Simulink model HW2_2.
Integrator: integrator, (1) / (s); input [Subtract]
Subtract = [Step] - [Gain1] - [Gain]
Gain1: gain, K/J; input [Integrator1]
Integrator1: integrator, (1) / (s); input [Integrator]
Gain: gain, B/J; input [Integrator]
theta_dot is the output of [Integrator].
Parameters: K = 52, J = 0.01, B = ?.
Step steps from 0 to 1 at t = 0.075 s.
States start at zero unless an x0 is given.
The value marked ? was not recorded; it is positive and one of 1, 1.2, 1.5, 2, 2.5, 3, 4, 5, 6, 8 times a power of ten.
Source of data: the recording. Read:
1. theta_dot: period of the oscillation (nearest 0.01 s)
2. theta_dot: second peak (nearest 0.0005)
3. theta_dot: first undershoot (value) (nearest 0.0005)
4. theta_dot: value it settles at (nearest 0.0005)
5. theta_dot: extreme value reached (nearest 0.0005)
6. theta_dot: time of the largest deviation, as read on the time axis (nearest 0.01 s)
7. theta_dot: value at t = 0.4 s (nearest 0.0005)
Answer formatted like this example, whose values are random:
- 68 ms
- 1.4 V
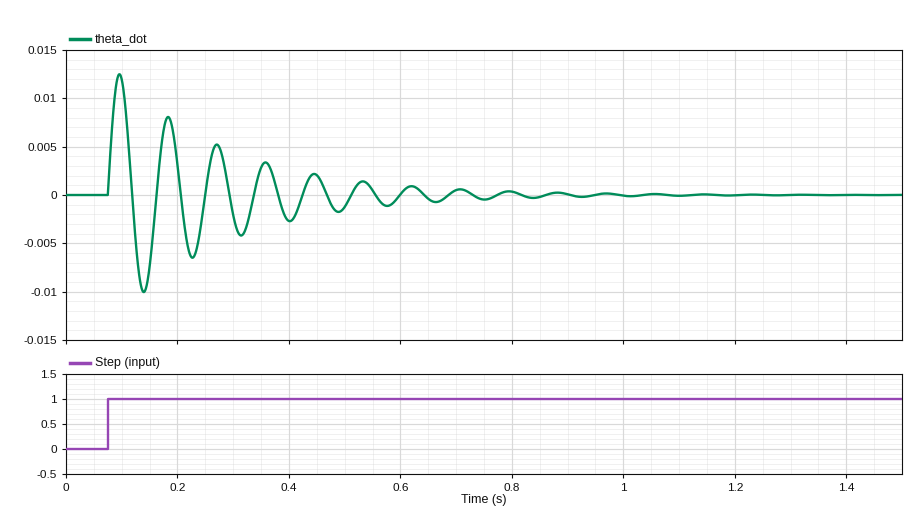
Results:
- 0.09 s
- 0.0080
- -0.0100
- 0.0000
- 0.0125
- 0.10 s
- -0.0025
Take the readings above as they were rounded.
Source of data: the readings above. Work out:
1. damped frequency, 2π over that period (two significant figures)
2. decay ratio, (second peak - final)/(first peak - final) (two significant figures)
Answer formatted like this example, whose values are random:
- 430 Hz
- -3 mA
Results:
- 70 rad/s
- 0.64
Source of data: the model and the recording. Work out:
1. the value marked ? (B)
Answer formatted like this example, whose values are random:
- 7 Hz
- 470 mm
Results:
- 0.1
